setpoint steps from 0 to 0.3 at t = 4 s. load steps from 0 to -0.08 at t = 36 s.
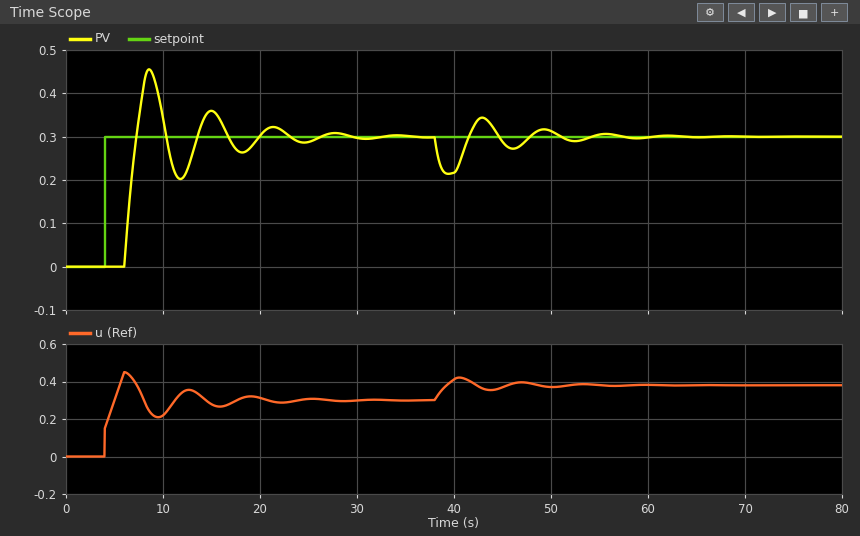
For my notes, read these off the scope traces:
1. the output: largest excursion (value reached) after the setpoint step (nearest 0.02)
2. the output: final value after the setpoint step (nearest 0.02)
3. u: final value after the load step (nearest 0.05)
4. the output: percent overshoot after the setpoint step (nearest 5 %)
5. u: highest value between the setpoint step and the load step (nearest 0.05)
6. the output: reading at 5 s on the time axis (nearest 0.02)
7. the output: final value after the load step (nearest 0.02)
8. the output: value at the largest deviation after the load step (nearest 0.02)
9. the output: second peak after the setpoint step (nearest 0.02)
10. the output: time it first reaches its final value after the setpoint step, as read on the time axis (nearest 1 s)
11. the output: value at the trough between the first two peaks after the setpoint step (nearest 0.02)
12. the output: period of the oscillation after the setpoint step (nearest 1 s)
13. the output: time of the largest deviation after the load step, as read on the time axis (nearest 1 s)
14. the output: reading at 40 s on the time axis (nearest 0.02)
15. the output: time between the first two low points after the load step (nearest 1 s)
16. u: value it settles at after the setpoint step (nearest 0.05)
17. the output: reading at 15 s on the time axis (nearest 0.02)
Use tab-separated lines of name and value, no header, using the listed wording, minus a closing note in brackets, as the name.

the output: largest excursion (value reached) after the setpoint step	0.46
the output: final value after the setpoint step	0.30
u: final value after the load step	0.40
the output: percent overshoot after the setpoint step	50 %
u: highest value between the setpoint step and the load step	0.45
the output: reading at 5 s on the time axis	0.00
the output: final value after the load step	0.30
the output: value at the largest deviation after the load step	0.22
the output: second peak after the setpoint step	0.36
the output: time it first reaches its final value after the setpoint step, as read on the time axis	7 s
the output: value at the trough between the first two peaks after the setpoint step	0.20
the output: period of the oscillation after the setpoint step	6 s
the output: time of the largest deviation after the load step, as read on the time axis	39 s
the output: reading at 40 s on the time axis	0.22
the output: time between the first two low points after the load step	7 s
u: value it settles at after the setpoint step	0.30
the output: reading at 15 s on the time axis	0.36
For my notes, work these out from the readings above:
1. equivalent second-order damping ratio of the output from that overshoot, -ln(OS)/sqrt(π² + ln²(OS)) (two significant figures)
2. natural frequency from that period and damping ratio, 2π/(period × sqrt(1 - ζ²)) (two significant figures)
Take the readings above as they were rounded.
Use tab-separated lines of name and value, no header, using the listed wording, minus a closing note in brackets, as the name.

equivalent second-order damping ratio of the output from that overshoot, -ln(OS)/sqrt(π² + ln²(OS))	0.22
natural frequency from that period and damping ratio, 2π/(period × sqrt(1 - ζ²))	1.1 rad/s
